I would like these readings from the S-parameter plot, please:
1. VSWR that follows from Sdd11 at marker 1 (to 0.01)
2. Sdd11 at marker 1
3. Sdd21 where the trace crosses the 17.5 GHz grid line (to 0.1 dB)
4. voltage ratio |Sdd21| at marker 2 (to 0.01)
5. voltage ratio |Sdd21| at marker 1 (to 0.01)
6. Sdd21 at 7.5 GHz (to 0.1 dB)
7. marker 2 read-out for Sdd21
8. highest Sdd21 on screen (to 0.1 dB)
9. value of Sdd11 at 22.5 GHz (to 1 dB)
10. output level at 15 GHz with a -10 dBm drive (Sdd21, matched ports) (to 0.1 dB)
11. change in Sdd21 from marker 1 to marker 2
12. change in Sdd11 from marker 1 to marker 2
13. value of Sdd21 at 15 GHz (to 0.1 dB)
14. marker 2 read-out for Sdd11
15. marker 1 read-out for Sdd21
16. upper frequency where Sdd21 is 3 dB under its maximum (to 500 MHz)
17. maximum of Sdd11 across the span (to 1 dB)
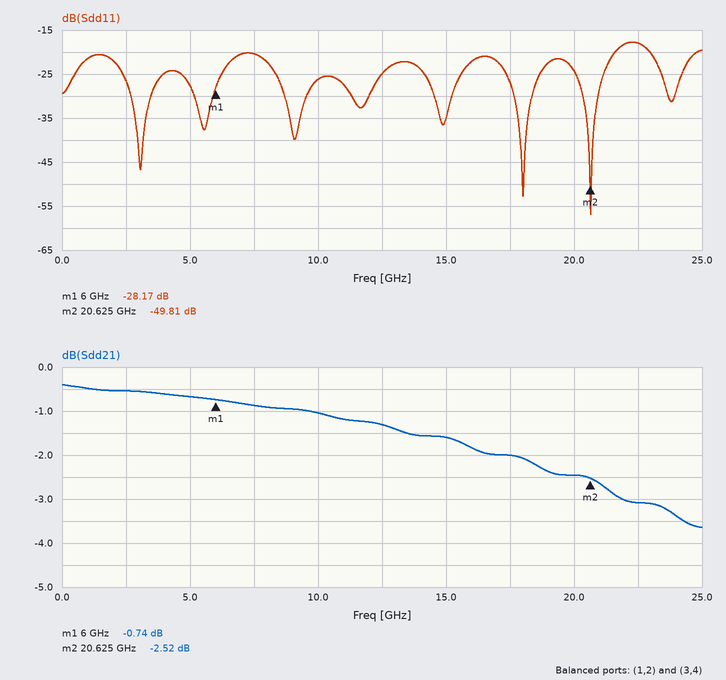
1.08
-28.17 dB
-2.0 dB
0.75
0.92
-0.9 dB
-2.52 dB
-0.4 dB
-18 dB
-11.6 dBm
-1.78 dB
-21.64 dB
-1.6 dB
-49.81 dB
-0.74 dB
24.0 GHz
-18 dB
